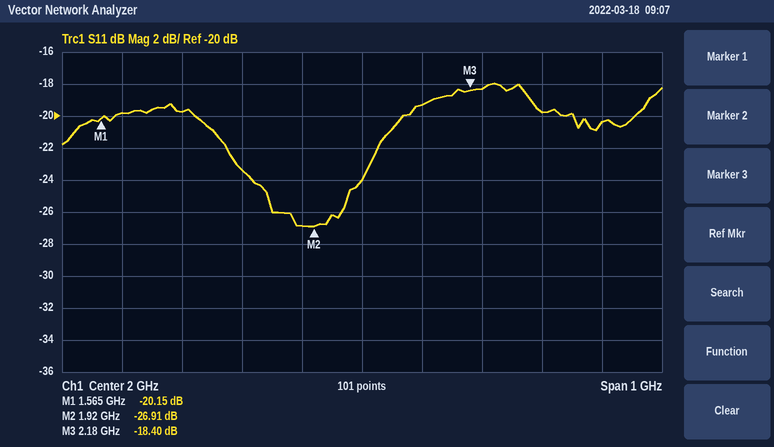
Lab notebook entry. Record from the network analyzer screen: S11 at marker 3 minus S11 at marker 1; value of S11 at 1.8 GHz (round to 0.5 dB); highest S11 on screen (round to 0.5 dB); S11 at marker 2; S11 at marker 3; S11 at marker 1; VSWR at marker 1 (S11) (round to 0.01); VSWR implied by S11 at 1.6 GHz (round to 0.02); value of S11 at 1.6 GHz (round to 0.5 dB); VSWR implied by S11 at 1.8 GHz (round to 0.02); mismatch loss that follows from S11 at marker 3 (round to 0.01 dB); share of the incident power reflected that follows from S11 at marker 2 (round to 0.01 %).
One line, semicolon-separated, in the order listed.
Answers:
1.75 dB; -23.5 dB; -18.0 dB; -26.91 dB; -18.40 dB; -20.15 dB; 1.22; 1.22; -20.0 dB; 1.14; 0.06 dB; 0.20 %
